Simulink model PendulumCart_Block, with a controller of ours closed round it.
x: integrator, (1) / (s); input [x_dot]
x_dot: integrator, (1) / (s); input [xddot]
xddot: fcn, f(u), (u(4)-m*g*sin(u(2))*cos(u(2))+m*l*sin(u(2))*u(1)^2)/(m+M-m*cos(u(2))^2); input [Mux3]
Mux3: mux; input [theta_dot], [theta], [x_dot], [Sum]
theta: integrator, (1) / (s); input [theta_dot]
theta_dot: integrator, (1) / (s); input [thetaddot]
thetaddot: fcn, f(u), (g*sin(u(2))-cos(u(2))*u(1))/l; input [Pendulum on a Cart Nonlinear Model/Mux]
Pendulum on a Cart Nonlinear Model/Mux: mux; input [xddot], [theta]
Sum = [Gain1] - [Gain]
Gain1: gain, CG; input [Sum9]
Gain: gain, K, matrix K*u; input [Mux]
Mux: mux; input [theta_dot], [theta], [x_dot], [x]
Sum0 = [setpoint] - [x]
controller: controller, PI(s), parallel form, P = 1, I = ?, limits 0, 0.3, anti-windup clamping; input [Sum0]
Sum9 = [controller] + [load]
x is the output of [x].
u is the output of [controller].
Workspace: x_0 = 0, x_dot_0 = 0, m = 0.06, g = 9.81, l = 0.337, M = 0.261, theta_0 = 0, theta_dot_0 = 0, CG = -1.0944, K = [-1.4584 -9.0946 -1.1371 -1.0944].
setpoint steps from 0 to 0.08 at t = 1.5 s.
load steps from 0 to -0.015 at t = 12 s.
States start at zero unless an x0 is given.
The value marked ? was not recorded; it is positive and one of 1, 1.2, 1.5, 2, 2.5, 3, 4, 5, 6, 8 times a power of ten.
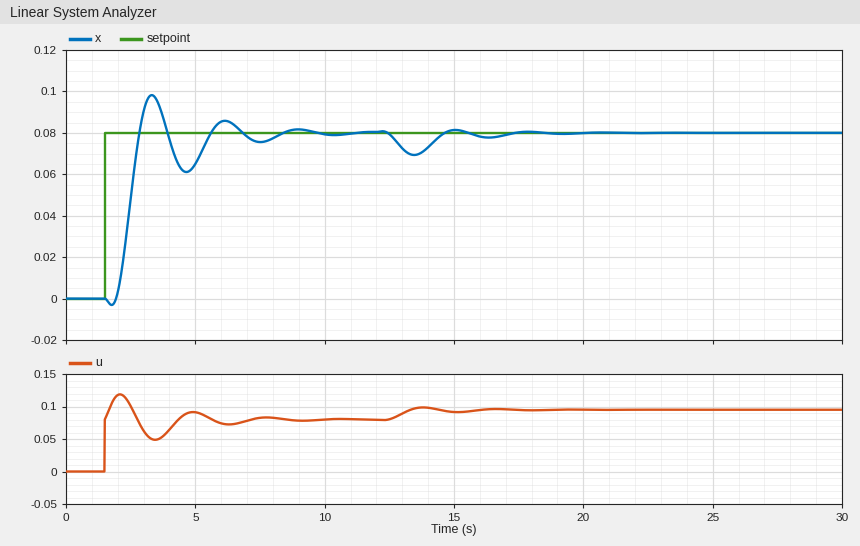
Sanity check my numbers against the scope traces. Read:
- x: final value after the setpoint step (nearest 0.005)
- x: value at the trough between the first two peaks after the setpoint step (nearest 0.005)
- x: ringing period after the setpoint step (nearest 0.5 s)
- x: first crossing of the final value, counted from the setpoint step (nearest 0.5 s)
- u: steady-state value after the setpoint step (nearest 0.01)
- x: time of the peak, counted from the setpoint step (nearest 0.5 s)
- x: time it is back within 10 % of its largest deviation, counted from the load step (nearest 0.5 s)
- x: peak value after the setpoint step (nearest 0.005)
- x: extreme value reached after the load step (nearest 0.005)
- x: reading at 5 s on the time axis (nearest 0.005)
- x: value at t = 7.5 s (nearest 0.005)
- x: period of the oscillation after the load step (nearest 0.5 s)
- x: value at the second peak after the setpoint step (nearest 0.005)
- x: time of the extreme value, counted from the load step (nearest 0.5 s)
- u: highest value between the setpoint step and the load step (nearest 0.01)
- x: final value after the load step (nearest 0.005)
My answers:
0.080
0.060
3.0 s
1.5 s
0.08
2.0 s
5.0 s
0.100
0.070
0.065
0.075
3.0 s
0.085
1.5 s
0.12
0.080
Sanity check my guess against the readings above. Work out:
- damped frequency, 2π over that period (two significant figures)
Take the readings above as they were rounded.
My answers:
2.1 rad/s
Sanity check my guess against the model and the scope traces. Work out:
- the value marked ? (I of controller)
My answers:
1
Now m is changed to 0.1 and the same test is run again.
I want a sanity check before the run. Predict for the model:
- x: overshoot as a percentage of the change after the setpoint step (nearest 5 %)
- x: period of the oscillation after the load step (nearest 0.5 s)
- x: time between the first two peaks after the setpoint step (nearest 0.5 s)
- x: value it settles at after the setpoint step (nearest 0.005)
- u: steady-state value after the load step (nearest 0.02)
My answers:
25 %
2.5 s
2.5 s
0.080
0.10
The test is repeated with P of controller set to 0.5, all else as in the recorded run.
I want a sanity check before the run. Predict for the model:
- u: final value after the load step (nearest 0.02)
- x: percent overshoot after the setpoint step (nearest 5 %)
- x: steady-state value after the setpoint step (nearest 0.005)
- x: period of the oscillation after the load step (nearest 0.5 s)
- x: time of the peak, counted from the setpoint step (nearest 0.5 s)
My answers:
0.10
20 %
0.080
4.0 s
2.5 s
